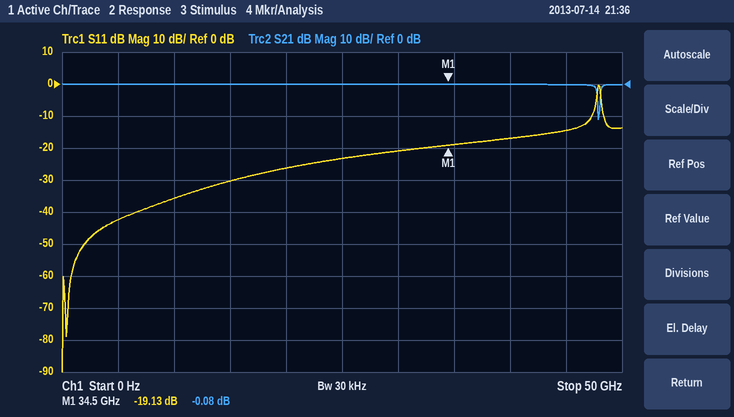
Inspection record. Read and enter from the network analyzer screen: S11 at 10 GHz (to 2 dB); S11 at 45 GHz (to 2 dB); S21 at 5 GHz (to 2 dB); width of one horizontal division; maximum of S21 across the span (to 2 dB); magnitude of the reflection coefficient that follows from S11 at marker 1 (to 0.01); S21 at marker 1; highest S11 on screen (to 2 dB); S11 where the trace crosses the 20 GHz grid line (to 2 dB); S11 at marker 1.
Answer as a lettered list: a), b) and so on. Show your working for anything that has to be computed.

a) -36 dB
b) -14 dB
c) 0 dB
d) 5 GHz
e) 0 dB
f) 10^(-19.13/20) ≈ 0.11
g) -0.08 dB
h) 0 dB
i) -26 dB
j) -19.13 dB
